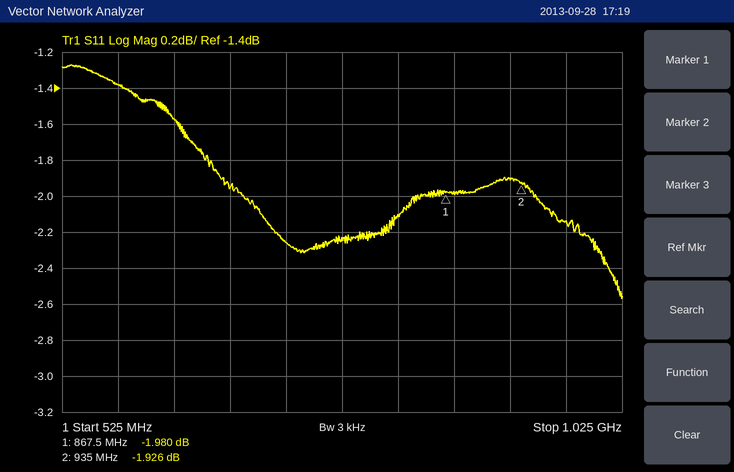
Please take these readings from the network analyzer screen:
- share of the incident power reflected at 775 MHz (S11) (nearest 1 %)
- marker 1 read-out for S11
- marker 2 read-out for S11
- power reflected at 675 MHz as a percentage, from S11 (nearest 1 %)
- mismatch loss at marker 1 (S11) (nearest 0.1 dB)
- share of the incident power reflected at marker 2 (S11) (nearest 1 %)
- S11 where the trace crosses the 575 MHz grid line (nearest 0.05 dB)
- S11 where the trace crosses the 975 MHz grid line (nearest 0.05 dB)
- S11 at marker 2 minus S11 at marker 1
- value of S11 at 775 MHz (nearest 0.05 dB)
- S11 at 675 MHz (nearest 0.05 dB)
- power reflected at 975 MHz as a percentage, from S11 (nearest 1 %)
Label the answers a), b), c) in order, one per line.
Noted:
a) 60 %
b) -1.980 dB
c) -1.926 dB
d) 64 %
e) 4.4 dB
f) 64 %
g) -1.40 dB
h) -2.15 dB
i) 0.054 dB
j) -2.25 dB
k) -1.95 dB
l) 61 %
